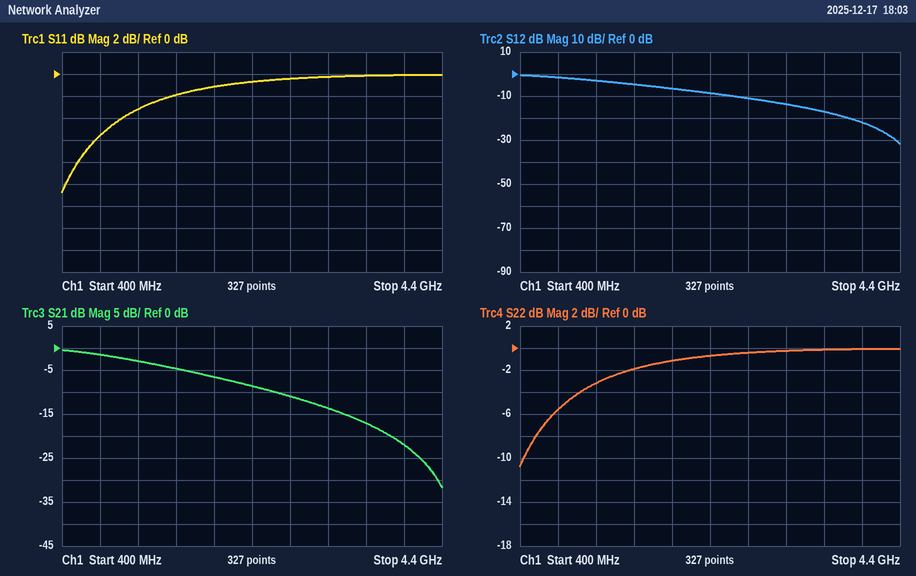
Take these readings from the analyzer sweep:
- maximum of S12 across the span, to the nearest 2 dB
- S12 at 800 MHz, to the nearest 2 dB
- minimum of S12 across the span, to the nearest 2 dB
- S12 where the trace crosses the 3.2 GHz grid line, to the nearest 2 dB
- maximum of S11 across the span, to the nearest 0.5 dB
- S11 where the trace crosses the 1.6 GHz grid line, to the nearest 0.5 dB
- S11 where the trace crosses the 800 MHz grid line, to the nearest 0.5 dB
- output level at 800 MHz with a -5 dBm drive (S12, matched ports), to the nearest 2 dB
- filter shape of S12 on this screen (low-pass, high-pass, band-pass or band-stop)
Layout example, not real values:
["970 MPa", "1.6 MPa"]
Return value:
["0 dB", "-2 dB", "-32 dB", "-14 dB", "0.0 dB", "-2.0 dB", "-5.5 dB", "-6 dBm", "low-pass"]
